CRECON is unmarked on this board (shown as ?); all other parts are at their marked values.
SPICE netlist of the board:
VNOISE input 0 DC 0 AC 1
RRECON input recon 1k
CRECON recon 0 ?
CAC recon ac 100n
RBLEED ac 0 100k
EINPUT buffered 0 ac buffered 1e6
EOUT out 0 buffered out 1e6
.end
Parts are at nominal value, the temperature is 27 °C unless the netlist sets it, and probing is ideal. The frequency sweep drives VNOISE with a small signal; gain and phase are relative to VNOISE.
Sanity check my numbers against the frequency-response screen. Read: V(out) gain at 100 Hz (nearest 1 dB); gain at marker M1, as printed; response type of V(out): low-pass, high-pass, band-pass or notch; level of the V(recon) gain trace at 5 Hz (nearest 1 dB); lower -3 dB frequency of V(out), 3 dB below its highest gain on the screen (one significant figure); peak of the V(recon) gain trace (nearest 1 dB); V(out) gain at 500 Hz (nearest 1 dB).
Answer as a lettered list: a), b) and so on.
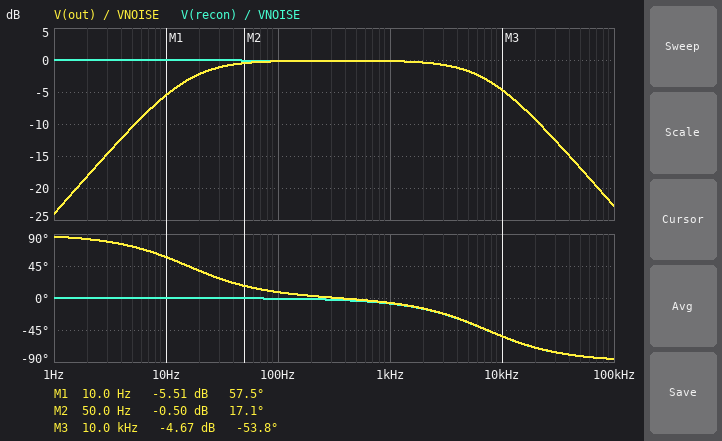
a) 0 dB
b) -5.51 dB
c) band-pass
d) 0 dB
e) 20 Hz
f) 0 dB
g) 0 dB
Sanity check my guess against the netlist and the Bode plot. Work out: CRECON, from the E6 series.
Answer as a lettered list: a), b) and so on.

a) 22 nF
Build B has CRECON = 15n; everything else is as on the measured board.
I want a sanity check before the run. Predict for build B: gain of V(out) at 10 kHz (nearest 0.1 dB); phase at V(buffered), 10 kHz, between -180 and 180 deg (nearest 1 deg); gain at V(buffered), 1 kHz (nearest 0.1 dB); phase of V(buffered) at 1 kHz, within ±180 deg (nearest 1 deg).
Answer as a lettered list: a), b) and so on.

a) -2.8 dB
b) -43 deg
c) -0.1 dB
d) -4 deg
